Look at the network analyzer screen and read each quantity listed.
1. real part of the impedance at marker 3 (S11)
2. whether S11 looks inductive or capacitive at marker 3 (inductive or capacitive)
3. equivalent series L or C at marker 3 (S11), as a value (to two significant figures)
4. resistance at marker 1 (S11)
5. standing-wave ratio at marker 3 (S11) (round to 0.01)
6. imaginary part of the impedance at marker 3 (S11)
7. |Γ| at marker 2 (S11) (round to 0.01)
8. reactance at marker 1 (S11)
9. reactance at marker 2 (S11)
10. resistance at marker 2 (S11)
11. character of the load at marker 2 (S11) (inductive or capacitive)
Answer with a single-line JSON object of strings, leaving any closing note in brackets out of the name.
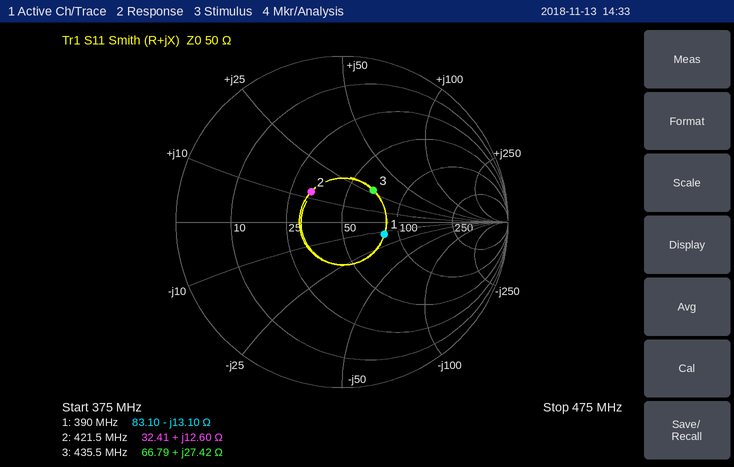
{"real part of the impedance at marker 3": "66.79 Ω", "whether S11 looks inductive or capacitive at marker 3": "inductive", "equivalent series L or C at marker 3 (S11), as a value": "10 nH", "resistance at marker 1": "83.10 Ω", "standing-wave ratio at marker 3 (S11)": "1.73", "imaginary part of the impedance at marker 3": "+27.42 Ω", "|Γ| at marker 2 (S11)": "0.26", "reactance at marker 1": "-13.10 Ω", "reactance at marker 2": "+12.60 Ω", "resistance at marker 2": "32.41 Ω", "character of the load at marker 2 (S11)": "inductive"}
